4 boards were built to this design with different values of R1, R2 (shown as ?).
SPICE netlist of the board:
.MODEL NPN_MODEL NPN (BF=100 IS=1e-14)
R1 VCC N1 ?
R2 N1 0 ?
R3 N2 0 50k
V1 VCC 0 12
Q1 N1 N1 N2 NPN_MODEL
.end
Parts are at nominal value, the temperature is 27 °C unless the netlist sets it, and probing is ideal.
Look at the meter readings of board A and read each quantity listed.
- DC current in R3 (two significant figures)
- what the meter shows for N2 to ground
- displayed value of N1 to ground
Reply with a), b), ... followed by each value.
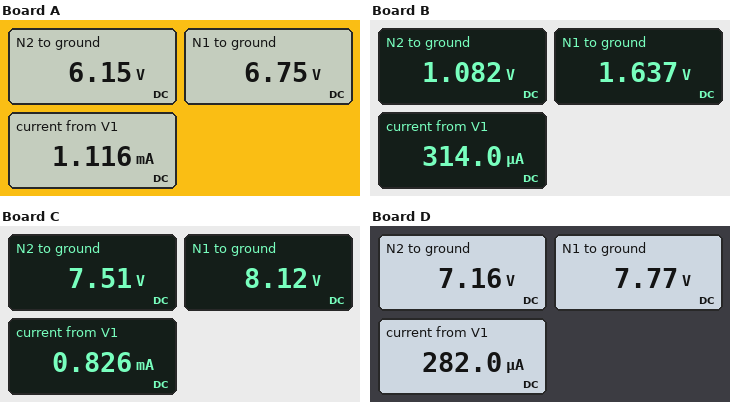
a) 120 µA
b) 6.15 V
c) 6.75 V
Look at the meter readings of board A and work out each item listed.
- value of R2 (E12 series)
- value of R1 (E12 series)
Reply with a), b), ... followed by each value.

a) 6.8 kΩ
b) 4.7 kΩ
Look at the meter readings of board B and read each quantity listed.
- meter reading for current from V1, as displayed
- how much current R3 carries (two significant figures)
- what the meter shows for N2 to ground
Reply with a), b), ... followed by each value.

a) 314.0 µA
b) 22 µA
c) 1.082 V
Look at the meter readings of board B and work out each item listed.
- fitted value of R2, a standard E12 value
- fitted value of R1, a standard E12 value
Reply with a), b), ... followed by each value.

a) 5.6 kΩ
b) 33 kΩ
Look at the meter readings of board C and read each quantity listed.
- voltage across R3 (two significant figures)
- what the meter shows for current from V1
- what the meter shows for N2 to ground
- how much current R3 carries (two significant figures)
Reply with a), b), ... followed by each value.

a) 7.5 V
b) 0.826 mA
c) 7.51 V
d) 150 µA
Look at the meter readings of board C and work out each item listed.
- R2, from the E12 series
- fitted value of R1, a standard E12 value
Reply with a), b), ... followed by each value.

a) 12 kΩ
b) 4.7 kΩ
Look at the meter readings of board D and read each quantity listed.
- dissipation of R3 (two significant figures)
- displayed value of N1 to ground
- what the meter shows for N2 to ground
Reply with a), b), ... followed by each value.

a) 1.0 mW
b) 7.77 V
c) 7.16 V
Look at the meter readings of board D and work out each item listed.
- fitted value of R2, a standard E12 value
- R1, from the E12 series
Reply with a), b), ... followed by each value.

a) 56 kΩ
b) 15 kΩ
